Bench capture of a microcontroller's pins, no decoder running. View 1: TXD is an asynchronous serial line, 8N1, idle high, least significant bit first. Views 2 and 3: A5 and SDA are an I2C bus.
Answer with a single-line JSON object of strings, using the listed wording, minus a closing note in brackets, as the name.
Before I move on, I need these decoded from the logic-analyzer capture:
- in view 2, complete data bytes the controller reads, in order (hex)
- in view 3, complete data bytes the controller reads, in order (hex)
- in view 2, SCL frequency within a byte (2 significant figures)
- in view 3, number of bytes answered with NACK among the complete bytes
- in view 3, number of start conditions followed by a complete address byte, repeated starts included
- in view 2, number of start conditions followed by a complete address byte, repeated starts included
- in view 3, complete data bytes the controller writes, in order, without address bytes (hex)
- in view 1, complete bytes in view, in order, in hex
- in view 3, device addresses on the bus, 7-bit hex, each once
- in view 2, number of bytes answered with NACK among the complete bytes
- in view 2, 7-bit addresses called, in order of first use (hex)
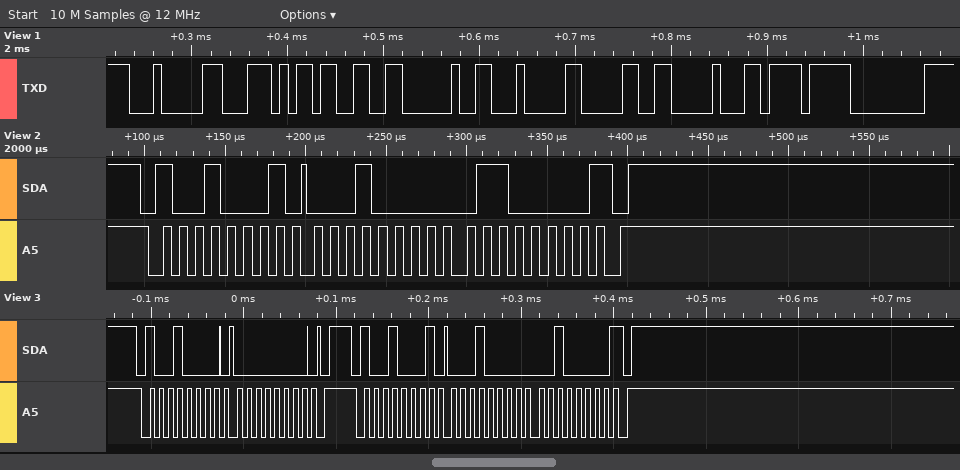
{"in view 2, complete data bytes the controller reads, in order": "10 60", "in view 3, complete data bytes the controller reads, in order": "10 20", "in view 2, SCL frequency within a byte": "100 kHz", "in view 3, number of bytes answered with NACK among the complete bytes": "1", "in view 3, number of start conditions followed by a complete address byte, repeated starts included": "2", "in view 2, number of start conditions followed by a complete address byte, repeated starts included": "1", "in view 3, complete data bytes the controller writes, in order, without address bytes": "00", "in view 1, complete bytes in view, in order, in hex": "04 5C 33 20 04 30 10 EF 00", "in view 3, device addresses on the bus, 7-bit hex, each once": "0x48", "in view 2, number of bytes answered with NACK among the complete bytes": "1", "in view 2, 7-bit addresses called, in order of first use": "0x48"}
